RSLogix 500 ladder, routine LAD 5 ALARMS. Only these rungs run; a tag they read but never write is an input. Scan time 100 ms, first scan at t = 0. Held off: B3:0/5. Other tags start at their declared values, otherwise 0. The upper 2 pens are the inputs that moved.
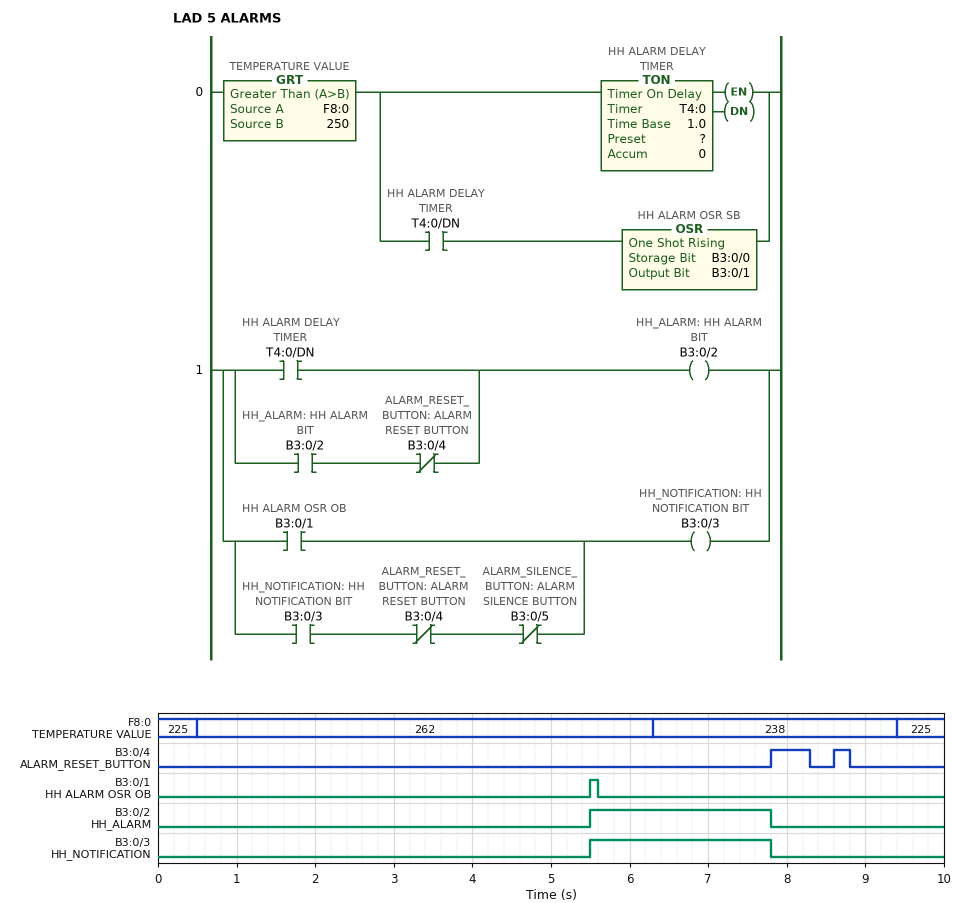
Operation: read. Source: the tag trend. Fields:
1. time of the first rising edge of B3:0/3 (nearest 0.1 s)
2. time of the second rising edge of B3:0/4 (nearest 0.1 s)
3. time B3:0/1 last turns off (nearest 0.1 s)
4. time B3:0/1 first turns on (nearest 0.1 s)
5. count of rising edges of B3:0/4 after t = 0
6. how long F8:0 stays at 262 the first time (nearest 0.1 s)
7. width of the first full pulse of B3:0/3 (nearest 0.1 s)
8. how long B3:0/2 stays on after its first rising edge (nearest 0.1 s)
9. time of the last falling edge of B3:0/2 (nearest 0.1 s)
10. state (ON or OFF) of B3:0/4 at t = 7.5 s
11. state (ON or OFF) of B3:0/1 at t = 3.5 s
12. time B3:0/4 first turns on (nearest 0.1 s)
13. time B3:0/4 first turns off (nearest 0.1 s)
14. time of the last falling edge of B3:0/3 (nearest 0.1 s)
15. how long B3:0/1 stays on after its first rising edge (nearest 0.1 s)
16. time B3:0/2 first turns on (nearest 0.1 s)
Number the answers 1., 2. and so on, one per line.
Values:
1. 5.5 s
2. 8.6 s
3. 5.6 s
4. 5.5 s
5. 2
6. 5.8 s
7. 2.3 s
8. 2.3 s
9. 7.8 s
10. OFF
11. OFF
12. 7.8 s
13. 8.3 s
14. 7.8 s
15. 0.1 s
16. 5.5 s
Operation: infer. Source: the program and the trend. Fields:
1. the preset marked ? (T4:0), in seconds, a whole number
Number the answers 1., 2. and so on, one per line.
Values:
1. 5 s
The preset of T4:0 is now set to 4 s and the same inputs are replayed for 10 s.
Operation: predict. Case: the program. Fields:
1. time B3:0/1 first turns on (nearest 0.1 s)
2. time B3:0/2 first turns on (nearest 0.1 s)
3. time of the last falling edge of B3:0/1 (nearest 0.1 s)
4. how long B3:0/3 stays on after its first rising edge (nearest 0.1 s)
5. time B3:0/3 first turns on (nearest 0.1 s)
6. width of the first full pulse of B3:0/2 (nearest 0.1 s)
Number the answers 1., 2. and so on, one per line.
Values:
1. 4.5 s
2. 4.5 s
3. 4.6 s
4. 3.3 s
5. 4.5 s
6. 3.3 s
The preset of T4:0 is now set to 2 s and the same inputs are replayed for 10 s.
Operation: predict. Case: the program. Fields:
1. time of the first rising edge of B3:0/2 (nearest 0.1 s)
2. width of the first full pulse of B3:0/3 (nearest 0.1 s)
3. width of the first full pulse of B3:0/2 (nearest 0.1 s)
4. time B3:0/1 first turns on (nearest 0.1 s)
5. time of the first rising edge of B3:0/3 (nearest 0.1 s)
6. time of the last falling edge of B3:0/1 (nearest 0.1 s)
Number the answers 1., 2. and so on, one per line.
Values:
1. 2.5 s
2. 5.3 s
3. 5.3 s
4. 2.5 s
5. 2.5 s
6. 2.6 s
